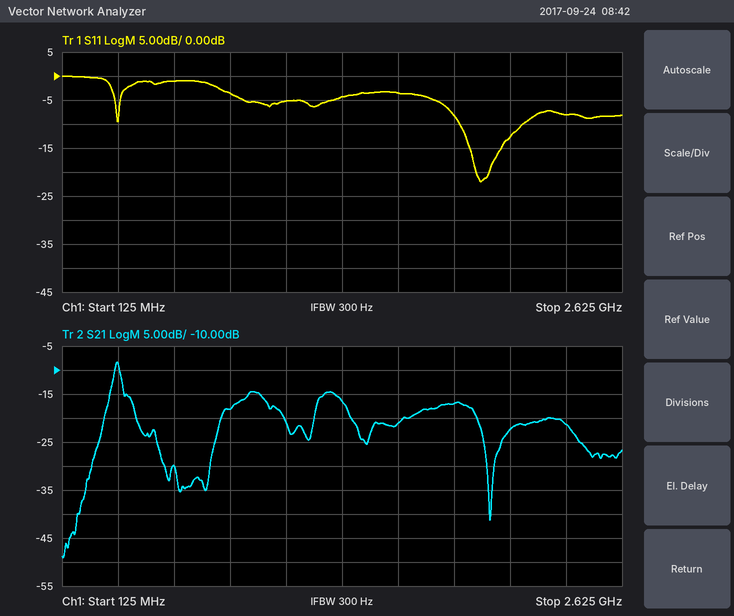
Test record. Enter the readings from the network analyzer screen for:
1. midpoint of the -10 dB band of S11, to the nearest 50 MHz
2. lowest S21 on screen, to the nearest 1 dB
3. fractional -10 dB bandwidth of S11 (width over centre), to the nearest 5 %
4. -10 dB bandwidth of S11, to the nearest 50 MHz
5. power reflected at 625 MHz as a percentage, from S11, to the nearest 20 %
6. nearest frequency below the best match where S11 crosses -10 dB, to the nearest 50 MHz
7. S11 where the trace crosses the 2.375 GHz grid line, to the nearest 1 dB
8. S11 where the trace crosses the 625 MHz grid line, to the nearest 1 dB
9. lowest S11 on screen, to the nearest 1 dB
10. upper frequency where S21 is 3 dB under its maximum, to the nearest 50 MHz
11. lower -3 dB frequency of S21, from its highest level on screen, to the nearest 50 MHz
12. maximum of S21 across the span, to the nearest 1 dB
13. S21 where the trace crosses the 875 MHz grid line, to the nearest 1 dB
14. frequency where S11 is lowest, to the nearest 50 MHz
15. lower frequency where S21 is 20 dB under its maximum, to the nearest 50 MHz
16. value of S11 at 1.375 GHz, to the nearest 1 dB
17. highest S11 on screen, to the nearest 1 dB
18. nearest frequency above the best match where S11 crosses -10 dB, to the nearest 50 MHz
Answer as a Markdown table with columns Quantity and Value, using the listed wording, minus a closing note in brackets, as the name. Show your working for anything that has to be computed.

| Quantity | Value |
|---|---|
| midpoint of the -10 dB band of S11, to the nearest 50 MHz | 2.05 GHz |
| lowest S21 on screen, to the nearest 1 dB | -49 dB |
| fractional -10 dB bandwidth of S11 (width over centre), to the nearest 5 % | 300 MHz / 2.05 GHz ≈ 15 % |
| -10 dB bandwidth of S11, to the nearest 50 MHz | 2.20 GHz − 1.90 GHz = 300 MHz |
| power reflected at 625 MHz as a percentage, from S11, to the nearest 20 % | 10^(-1/10) ≈ 79.4 %, so 80 % to the nearest 20 % |
| nearest frequency below the best match where S11 crosses -10 dB, to the nearest 50 MHz | 1.90 GHz |
| S11 where the trace crosses the 2.375 GHz grid line, to the nearest 1 dB | -8 dB |
| S11 where the trace crosses the 625 MHz grid line, to the nearest 1 dB | -1 dB |
| lowest S11 on screen, to the nearest 1 dB | -22 dB |
| upper frequency where S21 is 3 dB under its maximum, to the nearest 50 MHz | 400 MHz |
| lower -3 dB frequency of S21, from its highest level on screen, to the nearest 50 MHz | 350 MHz |
| maximum of S21 across the span, to the nearest 1 dB | -8 dB |
| S21 where the trace crosses the 875 MHz grid line, to the nearest 1 dB | -18 dB |
| frequency where S11 is lowest, to the nearest 50 MHz | 2.00 GHz |
| lower frequency where S21 is 20 dB under its maximum, to the nearest 50 MHz | 250 MHz |
| value of S11 at 1.375 GHz, to the nearest 1 dB | -4 dB |
| highest S11 on screen, to the nearest 1 dB | 0 dB |
| nearest frequency above the best match where S11 crosses -10 dB, to the nearest 50 MHz | 2.20 GHz |
